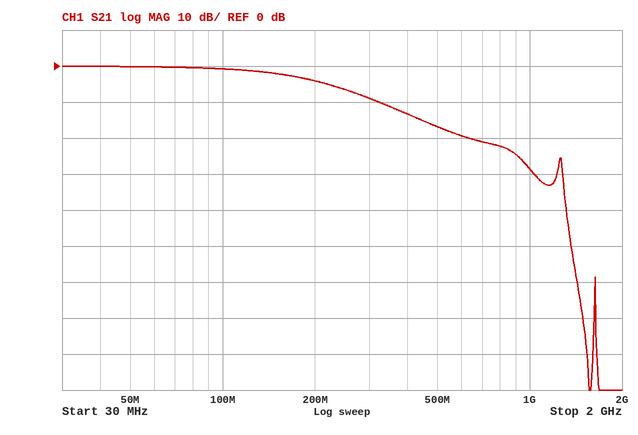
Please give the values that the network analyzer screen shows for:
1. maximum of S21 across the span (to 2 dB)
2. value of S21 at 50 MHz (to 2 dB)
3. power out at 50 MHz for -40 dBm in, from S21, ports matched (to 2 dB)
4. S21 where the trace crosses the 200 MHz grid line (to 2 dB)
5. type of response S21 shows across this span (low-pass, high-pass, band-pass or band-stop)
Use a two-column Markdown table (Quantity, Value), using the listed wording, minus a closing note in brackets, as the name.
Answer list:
| Quantity | Value |
|---|---|
| maximum of S21 across the span | 0 dB |
| value of S21 at 50 MHz | 0 dB |
| power out at 50 MHz for -40 dBm in, from S21, ports matched | -40 dBm |
| S21 where the trace crosses the 200 MHz grid line | -4 dB |
| type of response S21 shows across this span | low-pass |
